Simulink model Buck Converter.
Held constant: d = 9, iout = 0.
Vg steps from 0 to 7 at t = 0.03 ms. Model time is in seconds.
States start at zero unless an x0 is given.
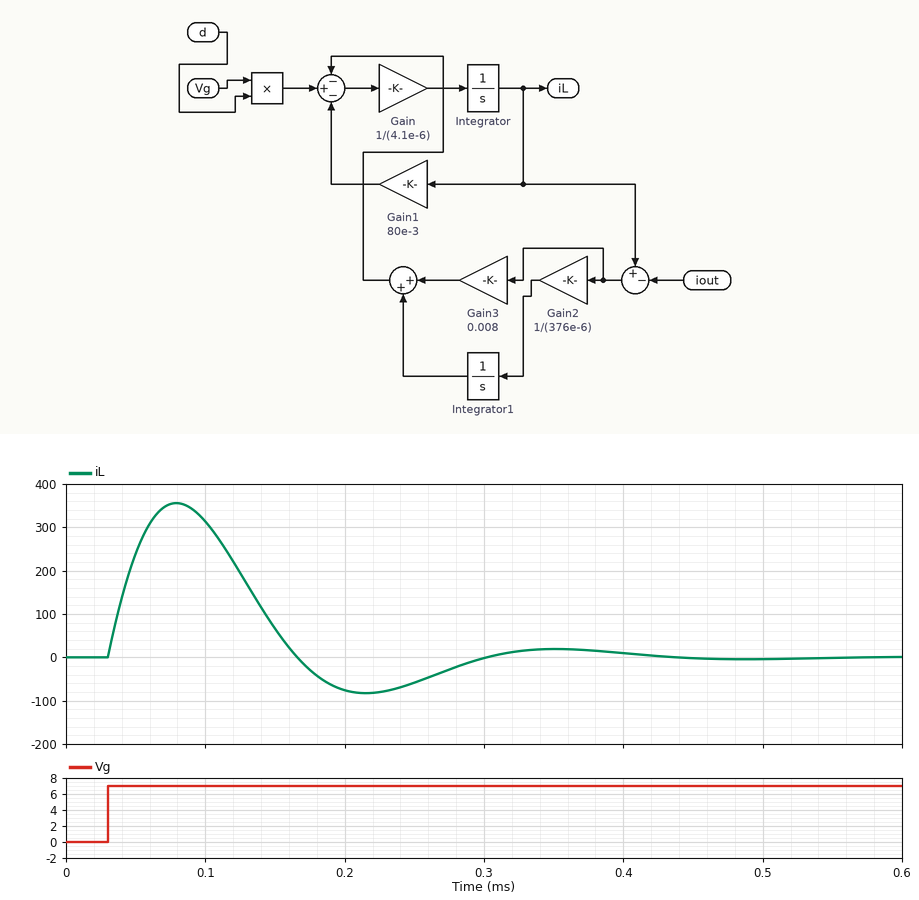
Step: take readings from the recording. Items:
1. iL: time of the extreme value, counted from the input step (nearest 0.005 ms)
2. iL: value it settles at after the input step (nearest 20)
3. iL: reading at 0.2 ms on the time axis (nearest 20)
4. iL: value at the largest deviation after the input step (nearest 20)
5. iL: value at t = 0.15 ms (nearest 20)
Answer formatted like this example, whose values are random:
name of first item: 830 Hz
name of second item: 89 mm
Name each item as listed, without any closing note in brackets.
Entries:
iL: time of the extreme value, counted from the input step: 0.050 ms
iL: value it settles at after the input step: 0
iL: reading at 0.2 ms on the time axis: -80
iL: value at the largest deviation after the input step: 360
iL: value at t = 0.15 ms: 60
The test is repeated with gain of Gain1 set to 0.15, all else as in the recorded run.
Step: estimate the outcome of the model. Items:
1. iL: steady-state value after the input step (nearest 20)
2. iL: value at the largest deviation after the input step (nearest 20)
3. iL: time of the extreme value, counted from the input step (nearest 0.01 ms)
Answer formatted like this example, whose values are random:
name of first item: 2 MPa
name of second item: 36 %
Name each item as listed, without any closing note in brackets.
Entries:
iL: steady-state value after the input step: 0
iL: value at the largest deviation after the input step: 260
iL: time of the extreme value, counted from the input step: 0.04 ms
